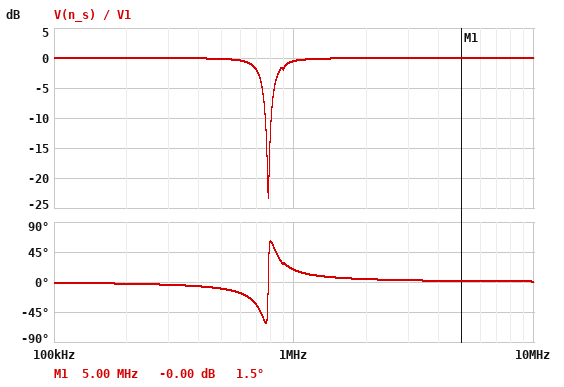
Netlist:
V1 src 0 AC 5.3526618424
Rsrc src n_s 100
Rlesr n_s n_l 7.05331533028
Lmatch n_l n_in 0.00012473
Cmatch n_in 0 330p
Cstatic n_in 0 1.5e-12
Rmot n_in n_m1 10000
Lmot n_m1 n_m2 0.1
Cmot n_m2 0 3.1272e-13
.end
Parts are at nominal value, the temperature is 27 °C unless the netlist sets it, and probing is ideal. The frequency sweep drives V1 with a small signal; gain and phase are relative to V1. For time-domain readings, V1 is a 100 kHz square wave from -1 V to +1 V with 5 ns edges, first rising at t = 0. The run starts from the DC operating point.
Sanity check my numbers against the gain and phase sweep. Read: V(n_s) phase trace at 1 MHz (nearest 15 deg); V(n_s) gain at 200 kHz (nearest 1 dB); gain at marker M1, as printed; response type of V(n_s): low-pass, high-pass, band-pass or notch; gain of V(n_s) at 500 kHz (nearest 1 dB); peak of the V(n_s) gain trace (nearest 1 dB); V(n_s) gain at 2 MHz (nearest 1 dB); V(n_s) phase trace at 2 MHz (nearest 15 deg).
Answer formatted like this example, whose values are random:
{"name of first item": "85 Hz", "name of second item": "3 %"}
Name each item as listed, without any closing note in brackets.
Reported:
{"V(n_s) phase trace at 1 MHz": "15 deg", "V(n_s) gain at 200 kHz": "0 dB", "gain at marker M1, as printed": "-0.00 dB", "response type of V(n_s): low-pass, high-pass, band-pass or notch": "notch", "gain of V(n_s) at 500 kHz": "0 dB", "peak of the V(n_s) gain trace": "0 dB", "V(n_s) gain at 2 MHz": "0 dB", "V(n_s) phase trace at 2 MHz": "0 deg"}
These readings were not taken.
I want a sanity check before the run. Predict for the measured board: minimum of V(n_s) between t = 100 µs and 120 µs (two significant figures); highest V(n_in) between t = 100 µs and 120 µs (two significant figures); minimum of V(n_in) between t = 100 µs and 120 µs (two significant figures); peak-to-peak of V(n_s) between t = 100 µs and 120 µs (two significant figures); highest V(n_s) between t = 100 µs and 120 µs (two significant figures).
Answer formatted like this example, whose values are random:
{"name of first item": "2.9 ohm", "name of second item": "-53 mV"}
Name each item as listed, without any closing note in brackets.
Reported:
{"minimum of V(n_s) between t = 100 µs and 120 µs": "-1.2 V", "highest V(n_in) between t = 100 µs and 120 µs": "2.4 V", "minimum of V(n_in) between t = 100 µs and 120 µs": "-2.4 V", "peak-to-peak of V(n_s) between t = 100 µs and 120 µs": "2.4 V", "highest V(n_s) between t = 100 µs and 120 µs": "1.2 V"}
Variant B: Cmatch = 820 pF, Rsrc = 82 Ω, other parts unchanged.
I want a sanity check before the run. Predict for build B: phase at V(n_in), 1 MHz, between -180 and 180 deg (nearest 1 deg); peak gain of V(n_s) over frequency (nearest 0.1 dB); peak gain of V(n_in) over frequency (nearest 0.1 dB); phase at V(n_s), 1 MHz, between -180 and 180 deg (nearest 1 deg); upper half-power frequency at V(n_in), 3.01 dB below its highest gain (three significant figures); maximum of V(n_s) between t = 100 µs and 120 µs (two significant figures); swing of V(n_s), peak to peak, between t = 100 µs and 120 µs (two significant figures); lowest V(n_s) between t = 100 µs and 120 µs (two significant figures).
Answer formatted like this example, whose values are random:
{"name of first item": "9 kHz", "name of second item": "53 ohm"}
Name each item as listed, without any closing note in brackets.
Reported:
{"phase at V(n_in), 1 MHz, between -180 and 180 deg": "-171 deg", "peak gain of V(n_s) over frequency": "0 dB", "peak gain of V(n_in) over frequency": "12.9 dB", "phase at V(n_s), 1 MHz, between -180 and 180 deg": "8 deg", "upper half-power frequency at V(n_in), 3.01 dB below its highest gain": "545 kHz", "maximum of V(n_s) between t = 100 µs and 120 µs": "1.3 V", "swing of V(n_s), peak to peak, between t = 100 µs and 120 µs": "2.6 V", "lowest V(n_s) between t = 100 µs and 120 µs": "-1.3 V"}
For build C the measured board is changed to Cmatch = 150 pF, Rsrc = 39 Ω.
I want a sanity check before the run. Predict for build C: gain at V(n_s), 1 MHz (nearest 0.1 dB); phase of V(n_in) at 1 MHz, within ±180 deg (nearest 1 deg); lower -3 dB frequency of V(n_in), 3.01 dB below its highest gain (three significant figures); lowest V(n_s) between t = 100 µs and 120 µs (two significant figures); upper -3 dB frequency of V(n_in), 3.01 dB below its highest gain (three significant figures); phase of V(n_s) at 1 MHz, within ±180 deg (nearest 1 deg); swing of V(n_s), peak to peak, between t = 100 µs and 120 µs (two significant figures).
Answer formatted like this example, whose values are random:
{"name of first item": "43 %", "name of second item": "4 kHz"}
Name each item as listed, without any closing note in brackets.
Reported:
{"gain at V(n_s), 1 MHz": "-0.1 dB", "phase of V(n_in) at 1 MHz, within ±180 deg": "-10 deg", "lower -3 dB frequency of V(n_in), 3.01 dB below its highest gain": "1.13 MHz", "lowest V(n_s) between t = 100 µs and 120 µs": "-1.1 V", "upper -3 dB frequency of V(n_in), 3.01 dB below its highest gain": "1.19 MHz", "phase of V(n_s) at 1 MHz, within ±180 deg": "-8 deg", "swing of V(n_s), peak to peak, between t = 100 µs and 120 µs": "2.1 V"}
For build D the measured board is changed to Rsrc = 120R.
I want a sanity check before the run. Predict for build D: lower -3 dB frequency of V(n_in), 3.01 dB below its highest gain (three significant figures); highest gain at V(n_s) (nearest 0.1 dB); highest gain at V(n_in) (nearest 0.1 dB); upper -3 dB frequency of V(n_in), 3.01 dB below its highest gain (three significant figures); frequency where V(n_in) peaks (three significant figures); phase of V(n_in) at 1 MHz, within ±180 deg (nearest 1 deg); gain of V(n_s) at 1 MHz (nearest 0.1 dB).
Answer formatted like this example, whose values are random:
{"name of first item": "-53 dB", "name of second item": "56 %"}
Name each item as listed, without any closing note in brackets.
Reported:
{"lower -3 dB frequency of V(n_in), 3.01 dB below its highest gain": "687 kHz", "highest gain at V(n_s)": "0 dB", "highest gain at V(n_in)": "13.7 dB", "upper -3 dB frequency of V(n_in), 3.01 dB below its highest gain": "848 kHz", "frequency where V(n_in) peaks": "773 kHz", "phase of V(n_in) at 1 MHz, within ±180 deg": "-157 deg", "gain of V(n_s) at 1 MHz": "-0.7 dB"}
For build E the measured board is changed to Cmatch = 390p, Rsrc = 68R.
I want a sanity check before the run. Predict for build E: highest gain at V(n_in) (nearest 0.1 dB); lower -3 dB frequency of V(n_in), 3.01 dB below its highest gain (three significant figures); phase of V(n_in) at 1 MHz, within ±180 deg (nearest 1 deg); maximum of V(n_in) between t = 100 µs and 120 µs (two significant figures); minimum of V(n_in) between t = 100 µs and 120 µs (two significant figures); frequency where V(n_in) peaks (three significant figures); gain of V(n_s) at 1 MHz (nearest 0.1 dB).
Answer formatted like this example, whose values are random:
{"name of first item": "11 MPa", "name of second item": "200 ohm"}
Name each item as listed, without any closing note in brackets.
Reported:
{"highest gain at V(n_in)": "17.5 dB", "lower -3 dB frequency of V(n_in), 3.01 dB below its highest gain": "667 kHz", "phase of V(n_in) at 1 MHz, within ±180 deg": "-169 deg", "maximum of V(n_in) between t = 100 µs and 120 µs": "3.0 V", "minimum of V(n_in) between t = 100 µs and 120 µs": "-3.0 V", "frequency where V(n_in) peaks": "716 kHz", "gain of V(n_s) at 1 MHz": "-0.2 dB"}
